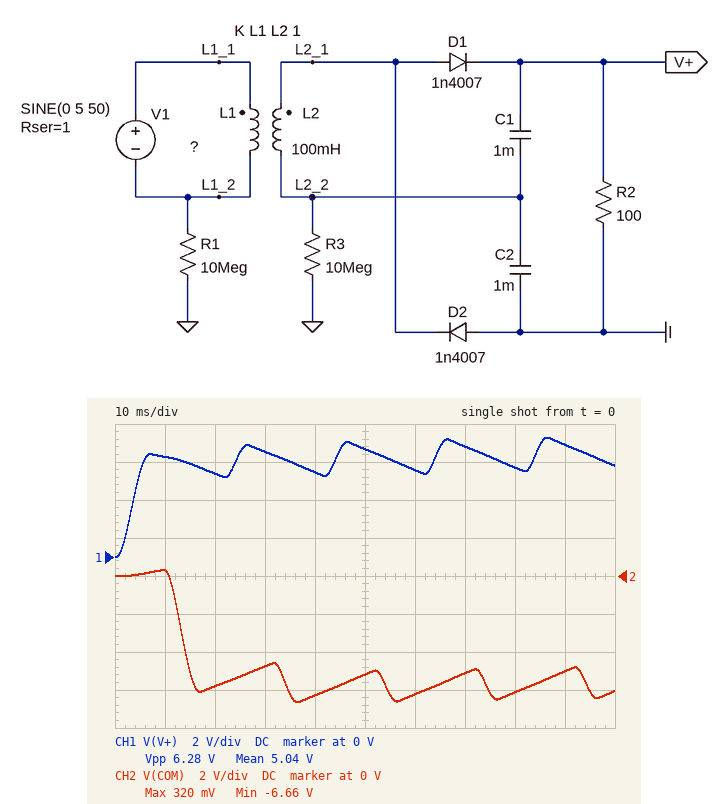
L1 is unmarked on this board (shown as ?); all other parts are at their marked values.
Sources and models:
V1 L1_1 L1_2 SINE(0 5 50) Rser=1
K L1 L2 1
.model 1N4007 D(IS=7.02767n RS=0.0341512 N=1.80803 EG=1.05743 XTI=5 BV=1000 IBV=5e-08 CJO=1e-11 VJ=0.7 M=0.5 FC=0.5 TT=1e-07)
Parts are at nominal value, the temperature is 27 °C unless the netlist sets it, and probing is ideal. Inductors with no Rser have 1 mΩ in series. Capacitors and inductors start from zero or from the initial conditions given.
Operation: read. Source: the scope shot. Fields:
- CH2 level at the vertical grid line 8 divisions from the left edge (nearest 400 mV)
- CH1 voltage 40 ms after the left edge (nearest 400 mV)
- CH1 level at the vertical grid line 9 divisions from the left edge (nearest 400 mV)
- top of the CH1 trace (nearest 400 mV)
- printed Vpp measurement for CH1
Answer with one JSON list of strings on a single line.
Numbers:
["-6.0 V", "4.4 V", "6.0 V", "6.4 V", "6.28 V"]
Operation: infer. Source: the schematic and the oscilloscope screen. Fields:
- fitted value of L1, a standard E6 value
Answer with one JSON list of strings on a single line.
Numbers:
["33 mH"]
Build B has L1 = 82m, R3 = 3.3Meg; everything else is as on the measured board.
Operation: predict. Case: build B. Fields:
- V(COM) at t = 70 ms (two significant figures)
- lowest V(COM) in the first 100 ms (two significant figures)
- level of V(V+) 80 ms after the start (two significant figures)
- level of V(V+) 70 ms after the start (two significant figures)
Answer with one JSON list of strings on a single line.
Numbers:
["-3.4 V", "-4.5 V", "3.2 V", "3.9 V"]
